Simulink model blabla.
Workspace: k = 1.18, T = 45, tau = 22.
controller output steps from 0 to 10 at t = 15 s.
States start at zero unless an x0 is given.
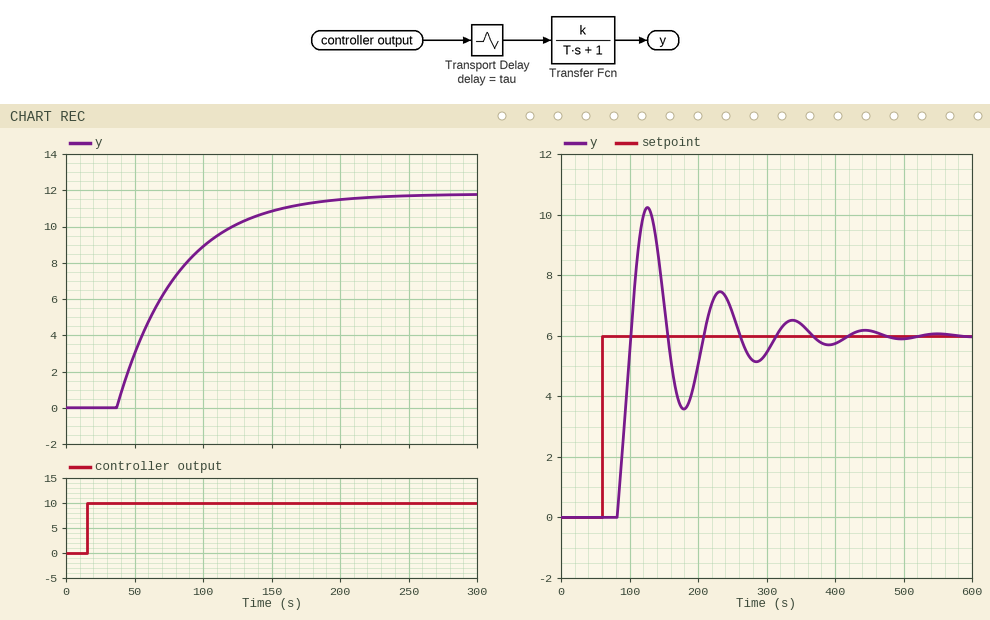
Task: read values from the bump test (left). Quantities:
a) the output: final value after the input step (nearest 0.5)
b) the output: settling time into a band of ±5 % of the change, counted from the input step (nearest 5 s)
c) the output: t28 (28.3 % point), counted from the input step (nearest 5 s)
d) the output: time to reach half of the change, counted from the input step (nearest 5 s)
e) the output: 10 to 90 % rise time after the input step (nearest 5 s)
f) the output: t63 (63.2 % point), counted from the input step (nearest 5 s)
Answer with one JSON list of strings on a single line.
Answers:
["12.0", "155 s", "35 s", "55 s", "100 s", "65 s"]
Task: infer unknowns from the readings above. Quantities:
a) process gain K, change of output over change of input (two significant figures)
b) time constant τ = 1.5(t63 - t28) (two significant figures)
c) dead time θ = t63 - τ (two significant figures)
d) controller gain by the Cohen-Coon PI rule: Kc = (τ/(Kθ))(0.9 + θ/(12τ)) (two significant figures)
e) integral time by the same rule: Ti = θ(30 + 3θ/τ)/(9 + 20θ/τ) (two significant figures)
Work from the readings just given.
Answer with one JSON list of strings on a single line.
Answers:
["1.2", "45 s", "20 s", "1.8", "35 s"]
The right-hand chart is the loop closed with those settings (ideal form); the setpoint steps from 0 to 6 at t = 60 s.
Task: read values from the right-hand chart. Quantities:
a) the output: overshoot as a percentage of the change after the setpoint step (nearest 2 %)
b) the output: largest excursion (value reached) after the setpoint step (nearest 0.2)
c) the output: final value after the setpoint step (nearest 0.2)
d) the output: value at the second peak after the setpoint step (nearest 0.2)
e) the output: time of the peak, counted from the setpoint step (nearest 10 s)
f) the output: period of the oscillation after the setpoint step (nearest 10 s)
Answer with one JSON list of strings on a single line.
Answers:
["70 %", "10.2", "6.0", "7.4", "70 s", "110 s"]
